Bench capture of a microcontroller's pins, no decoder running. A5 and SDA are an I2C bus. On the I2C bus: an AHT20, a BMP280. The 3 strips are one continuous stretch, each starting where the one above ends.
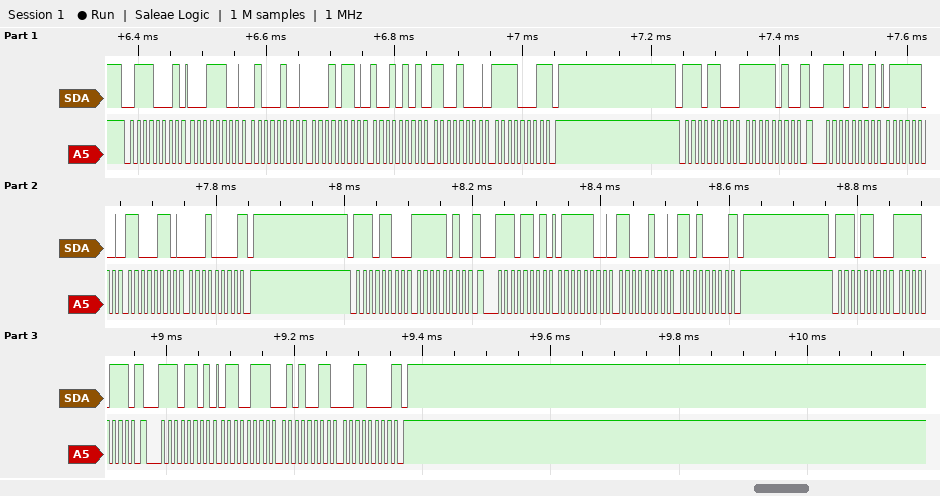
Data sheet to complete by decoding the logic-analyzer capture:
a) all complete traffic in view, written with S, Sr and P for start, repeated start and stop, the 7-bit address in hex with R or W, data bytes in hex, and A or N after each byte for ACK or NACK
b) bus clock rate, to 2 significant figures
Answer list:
S 38R A 1C A 44 A 16 A 95 A C8 A F1 N P S 76W A FA A Sr 76R A 7C A C6 A 10 N P S 76W A FA A Sr 76R A 7C A C4 A D0 N P S 76W A F7 A Sr 76R A 67 A 53 A 30 N P
100 kHz
